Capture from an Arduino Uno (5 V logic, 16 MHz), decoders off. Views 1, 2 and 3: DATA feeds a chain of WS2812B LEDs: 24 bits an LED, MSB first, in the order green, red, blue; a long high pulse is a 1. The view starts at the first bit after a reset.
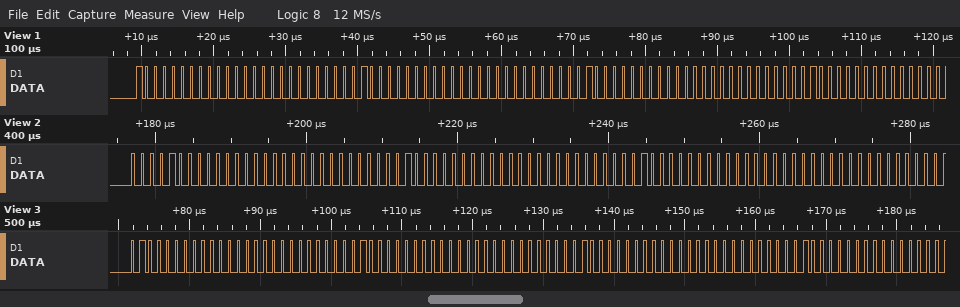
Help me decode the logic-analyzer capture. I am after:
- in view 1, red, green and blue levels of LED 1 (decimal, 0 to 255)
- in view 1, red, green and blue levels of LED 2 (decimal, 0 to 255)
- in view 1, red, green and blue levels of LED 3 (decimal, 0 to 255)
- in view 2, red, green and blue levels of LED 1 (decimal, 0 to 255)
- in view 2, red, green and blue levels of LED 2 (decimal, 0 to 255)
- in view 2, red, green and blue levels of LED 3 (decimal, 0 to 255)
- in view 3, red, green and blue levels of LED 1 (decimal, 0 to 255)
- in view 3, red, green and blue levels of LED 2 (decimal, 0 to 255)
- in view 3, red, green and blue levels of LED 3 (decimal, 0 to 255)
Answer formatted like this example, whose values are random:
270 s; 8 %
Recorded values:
0, 128, 0; 0, 64, 0; 0, 32, 0; 0, 8, 0; 0, 4, 0; 0, 2, 0; 0, 64, 0; 0, 32, 0; 0, 16, 0
